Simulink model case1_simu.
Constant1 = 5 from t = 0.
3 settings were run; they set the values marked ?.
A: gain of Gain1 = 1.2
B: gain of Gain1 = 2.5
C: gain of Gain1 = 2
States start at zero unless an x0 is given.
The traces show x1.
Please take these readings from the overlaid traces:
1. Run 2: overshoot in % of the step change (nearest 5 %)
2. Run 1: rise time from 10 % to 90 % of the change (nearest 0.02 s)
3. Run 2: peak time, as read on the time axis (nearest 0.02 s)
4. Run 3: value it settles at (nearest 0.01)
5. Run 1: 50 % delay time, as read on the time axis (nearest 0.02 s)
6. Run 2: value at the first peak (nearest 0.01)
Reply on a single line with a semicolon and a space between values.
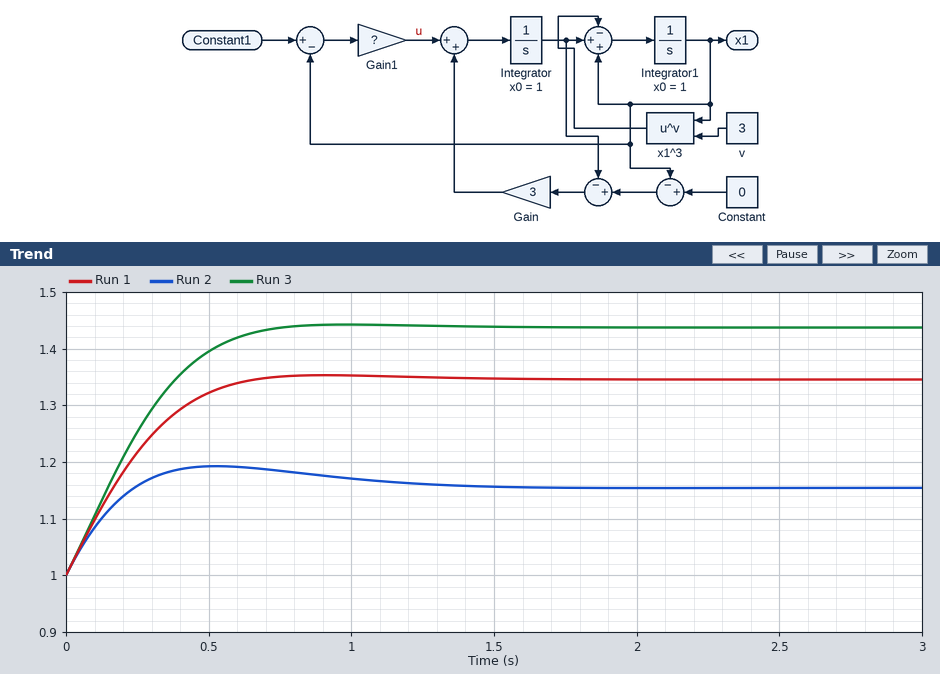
25 %; 0.42 s; 0.52 s; 1.44; 0.18 s; 1.19
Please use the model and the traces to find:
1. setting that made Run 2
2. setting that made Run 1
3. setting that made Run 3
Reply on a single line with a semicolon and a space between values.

A; C; B
